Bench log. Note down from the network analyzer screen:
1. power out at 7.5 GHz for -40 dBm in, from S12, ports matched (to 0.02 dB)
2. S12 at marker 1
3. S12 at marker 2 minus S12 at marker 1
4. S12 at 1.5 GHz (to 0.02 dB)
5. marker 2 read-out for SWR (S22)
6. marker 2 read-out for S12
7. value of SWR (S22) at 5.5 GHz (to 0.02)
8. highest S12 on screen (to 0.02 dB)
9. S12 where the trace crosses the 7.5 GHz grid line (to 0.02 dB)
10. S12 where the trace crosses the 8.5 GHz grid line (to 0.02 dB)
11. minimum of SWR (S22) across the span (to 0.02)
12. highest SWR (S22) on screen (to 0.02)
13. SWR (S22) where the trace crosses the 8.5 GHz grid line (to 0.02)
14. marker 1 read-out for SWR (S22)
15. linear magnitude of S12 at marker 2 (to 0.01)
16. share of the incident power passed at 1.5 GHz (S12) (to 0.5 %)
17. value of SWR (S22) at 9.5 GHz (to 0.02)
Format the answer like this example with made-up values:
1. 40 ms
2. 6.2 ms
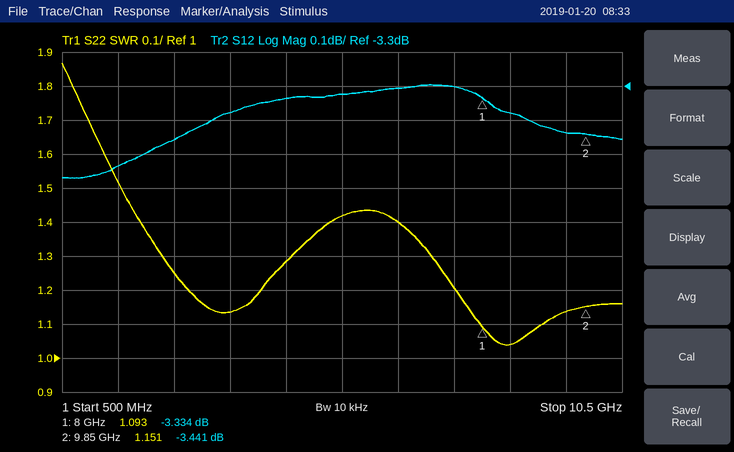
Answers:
1. -43.30 dBm
2. -3.334 dB
3. -0.107 dB
4. -3.54 dB
5. 1.151
6. -3.441 dB
7. 1.42
8. -3.30 dB
9. -3.30 dB
10. -3.38 dB
11. 1.04
12. 1.86
13. 1.04
14. 1.093
15. 0.67
16. 44.5 %
17. 1.14
